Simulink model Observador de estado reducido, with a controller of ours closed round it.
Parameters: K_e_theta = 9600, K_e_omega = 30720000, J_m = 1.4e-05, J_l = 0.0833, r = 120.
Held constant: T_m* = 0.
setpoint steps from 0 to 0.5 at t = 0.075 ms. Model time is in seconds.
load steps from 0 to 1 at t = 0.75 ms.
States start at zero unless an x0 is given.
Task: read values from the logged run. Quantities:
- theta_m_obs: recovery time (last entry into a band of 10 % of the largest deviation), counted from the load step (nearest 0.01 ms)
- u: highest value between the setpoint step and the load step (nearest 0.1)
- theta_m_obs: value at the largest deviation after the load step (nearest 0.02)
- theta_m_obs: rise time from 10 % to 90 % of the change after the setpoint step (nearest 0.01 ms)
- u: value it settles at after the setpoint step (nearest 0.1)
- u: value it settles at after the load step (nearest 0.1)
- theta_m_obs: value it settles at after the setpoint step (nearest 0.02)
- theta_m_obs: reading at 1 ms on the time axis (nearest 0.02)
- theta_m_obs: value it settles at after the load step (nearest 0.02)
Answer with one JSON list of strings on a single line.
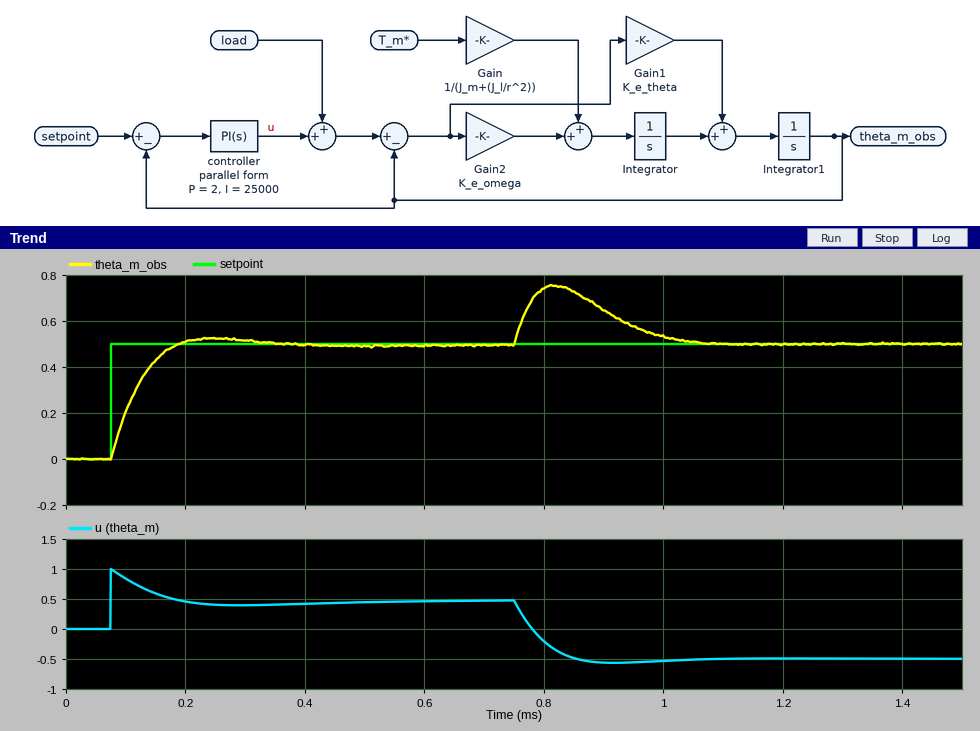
["0.26 ms", "1.0", "0.76", "0.08 ms", "0.5", "-0.5", "0.50", "0.54", "0.50"]
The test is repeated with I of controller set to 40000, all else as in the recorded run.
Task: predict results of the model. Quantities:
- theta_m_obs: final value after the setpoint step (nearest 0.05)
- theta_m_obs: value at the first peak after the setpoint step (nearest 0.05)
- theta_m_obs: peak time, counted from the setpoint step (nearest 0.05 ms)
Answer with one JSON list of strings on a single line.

["0.50", "0.55", "0.15 ms"]
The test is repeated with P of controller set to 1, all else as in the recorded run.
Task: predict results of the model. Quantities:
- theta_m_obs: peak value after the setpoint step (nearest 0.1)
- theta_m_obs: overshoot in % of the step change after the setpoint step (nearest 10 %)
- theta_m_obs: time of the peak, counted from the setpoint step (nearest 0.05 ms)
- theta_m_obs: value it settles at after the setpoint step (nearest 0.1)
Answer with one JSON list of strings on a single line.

["0.6", "20 %", "0.20 ms", "0.5"]
